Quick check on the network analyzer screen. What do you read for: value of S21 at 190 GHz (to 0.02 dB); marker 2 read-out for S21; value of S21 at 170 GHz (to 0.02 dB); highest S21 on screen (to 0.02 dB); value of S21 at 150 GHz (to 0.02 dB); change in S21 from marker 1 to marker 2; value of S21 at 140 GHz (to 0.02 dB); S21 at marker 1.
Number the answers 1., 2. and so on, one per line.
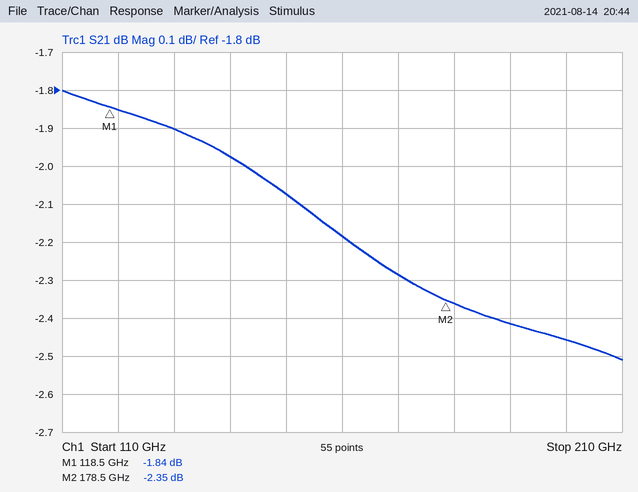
1. -2.42 dB
2. -2.35 dB
3. -2.28 dB
4. -1.80 dB
5. -2.08 dB
6. -0.51 dB
7. -1.98 dB
8. -1.84 dB
